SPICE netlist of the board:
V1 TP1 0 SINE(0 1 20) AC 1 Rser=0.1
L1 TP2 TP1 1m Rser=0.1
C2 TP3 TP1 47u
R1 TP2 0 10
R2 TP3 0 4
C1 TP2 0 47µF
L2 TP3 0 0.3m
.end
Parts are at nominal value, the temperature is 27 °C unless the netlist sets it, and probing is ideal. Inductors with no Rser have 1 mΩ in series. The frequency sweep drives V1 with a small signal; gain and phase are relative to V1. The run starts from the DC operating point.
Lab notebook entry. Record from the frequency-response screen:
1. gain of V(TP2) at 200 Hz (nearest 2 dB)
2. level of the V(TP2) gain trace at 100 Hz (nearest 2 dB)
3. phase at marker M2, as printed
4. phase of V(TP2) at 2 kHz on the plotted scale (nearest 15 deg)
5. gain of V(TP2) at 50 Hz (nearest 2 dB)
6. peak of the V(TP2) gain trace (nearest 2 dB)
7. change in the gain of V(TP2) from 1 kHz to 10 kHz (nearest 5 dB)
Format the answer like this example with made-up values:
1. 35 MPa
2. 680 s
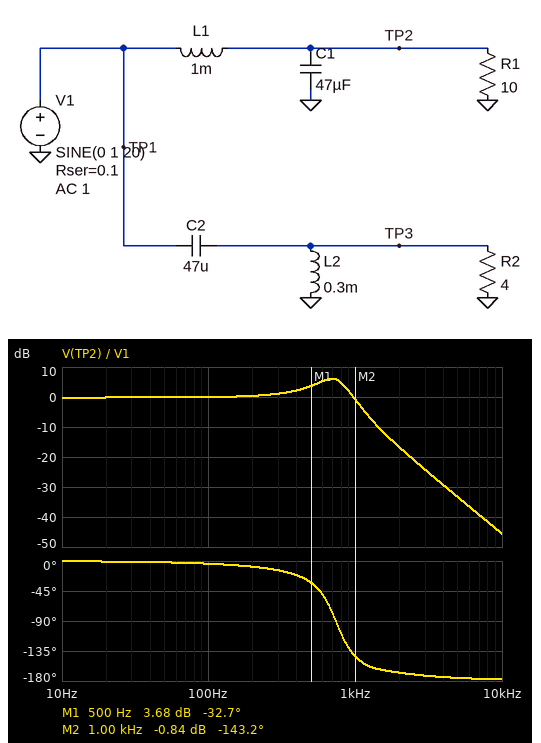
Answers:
1. 0 dB
2. 0 dB
3. -143.2 deg
4. -165 deg
5. 0 dB
6. 6 dB
7. -45 dB
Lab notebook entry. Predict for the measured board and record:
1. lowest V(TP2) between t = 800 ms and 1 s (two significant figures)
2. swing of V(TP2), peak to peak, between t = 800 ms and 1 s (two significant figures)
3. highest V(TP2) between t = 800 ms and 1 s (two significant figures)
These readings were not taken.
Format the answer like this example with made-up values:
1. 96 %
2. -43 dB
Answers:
1. -980 mV
2. 2.0 V
3. 980 mV
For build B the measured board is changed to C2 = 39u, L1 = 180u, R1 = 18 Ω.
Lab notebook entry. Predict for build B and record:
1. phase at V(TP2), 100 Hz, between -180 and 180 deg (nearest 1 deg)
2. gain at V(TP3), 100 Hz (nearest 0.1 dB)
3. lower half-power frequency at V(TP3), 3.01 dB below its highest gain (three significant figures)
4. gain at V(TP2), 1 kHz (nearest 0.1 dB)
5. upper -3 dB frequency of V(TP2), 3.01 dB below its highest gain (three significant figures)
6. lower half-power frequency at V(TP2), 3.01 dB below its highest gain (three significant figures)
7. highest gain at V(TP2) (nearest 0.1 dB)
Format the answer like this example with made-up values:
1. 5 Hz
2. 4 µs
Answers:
1. -1 deg
2. -46.7 dB
3. 1.18 kHz
4. 3.1 dB
5. 1.89 kHz
6. 1.53 kHz
7. 13.1 dB
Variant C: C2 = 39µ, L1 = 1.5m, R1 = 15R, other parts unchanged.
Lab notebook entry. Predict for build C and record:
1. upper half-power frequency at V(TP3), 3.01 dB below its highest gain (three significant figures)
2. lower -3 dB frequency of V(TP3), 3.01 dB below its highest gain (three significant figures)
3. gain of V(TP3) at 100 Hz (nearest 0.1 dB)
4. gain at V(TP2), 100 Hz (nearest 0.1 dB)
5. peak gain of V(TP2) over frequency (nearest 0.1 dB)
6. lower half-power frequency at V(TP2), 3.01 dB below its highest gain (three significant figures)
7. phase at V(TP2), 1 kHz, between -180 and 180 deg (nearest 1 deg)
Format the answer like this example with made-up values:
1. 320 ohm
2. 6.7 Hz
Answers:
1. 5.58 kHz
2. 1.22 kHz
3. -46.7 dB
4. 0.1 dB
5. 7.8 dB
6. 433 Hz
7. -161 deg
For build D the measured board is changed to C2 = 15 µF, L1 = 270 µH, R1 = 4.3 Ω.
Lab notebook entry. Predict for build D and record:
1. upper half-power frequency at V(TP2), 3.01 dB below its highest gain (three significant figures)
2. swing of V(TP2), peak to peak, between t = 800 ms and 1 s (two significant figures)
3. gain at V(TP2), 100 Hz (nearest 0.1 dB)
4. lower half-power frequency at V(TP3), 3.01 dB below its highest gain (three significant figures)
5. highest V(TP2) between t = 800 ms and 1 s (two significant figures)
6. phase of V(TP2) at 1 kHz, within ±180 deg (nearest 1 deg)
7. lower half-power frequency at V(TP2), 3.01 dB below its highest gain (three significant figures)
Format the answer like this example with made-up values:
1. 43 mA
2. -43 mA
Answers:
1. 1.71 kHz
2. 1.9 V
3. -0.4 dB
4. 2.08 kHz
5. 960 mV
6. -40 deg
7. 657 Hz
